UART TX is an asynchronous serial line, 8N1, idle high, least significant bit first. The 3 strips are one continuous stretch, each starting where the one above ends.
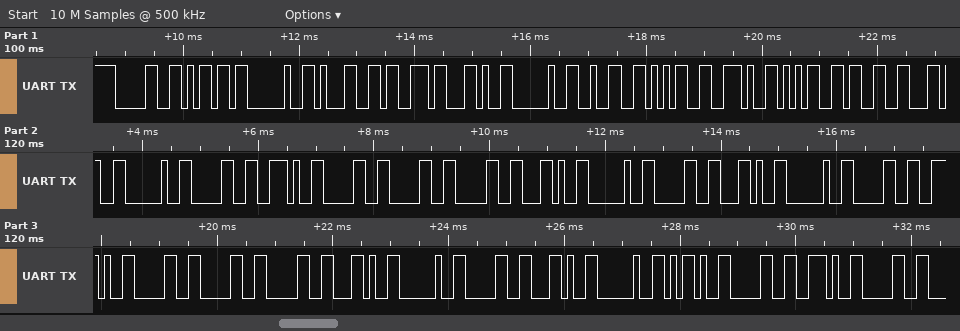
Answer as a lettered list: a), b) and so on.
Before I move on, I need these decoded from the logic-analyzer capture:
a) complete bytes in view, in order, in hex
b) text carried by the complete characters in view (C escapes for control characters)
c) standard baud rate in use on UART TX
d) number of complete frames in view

a) 0x30 0x6D 0x20 0x31 0x73 0x2C 0x20 0x32 0x35 0x2E 0x35 0x33 0x2C 0x20 0x30 0x2E 0x30 0x30 0x30 0x2C 0x20 0x30 0x2C 0x20 0x30 0x2E 0x30 0x30 0x30 0x2C 0x20 0x30 0x2C 0x20 0x2D 0x30 0x2E 0x30
b) "0m 1s, 25.53, 0.000, 0, 0.000, 0, -0.0"
c) 9600 baud
d) 38
